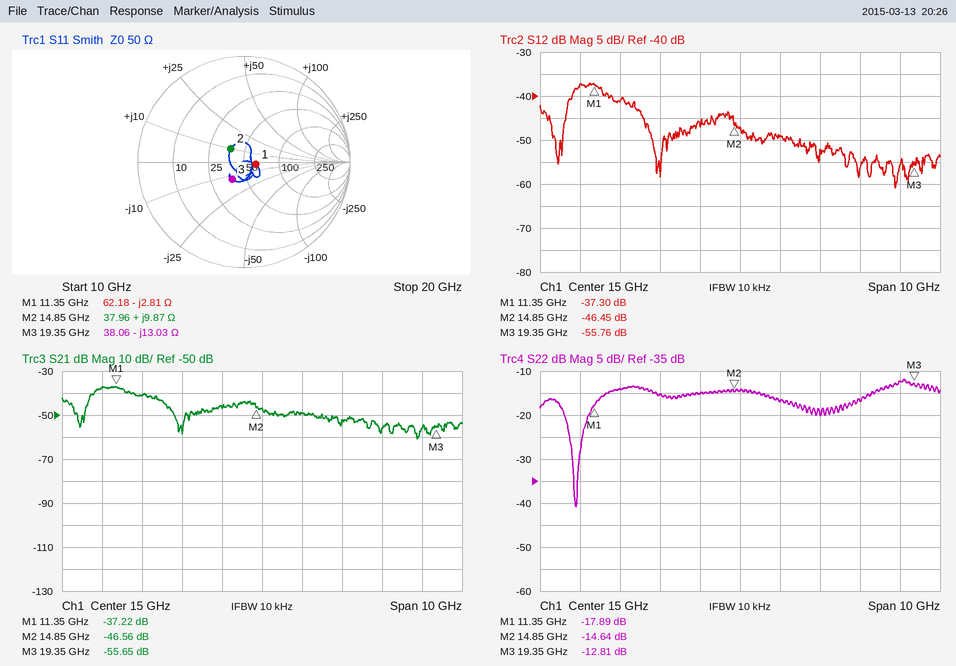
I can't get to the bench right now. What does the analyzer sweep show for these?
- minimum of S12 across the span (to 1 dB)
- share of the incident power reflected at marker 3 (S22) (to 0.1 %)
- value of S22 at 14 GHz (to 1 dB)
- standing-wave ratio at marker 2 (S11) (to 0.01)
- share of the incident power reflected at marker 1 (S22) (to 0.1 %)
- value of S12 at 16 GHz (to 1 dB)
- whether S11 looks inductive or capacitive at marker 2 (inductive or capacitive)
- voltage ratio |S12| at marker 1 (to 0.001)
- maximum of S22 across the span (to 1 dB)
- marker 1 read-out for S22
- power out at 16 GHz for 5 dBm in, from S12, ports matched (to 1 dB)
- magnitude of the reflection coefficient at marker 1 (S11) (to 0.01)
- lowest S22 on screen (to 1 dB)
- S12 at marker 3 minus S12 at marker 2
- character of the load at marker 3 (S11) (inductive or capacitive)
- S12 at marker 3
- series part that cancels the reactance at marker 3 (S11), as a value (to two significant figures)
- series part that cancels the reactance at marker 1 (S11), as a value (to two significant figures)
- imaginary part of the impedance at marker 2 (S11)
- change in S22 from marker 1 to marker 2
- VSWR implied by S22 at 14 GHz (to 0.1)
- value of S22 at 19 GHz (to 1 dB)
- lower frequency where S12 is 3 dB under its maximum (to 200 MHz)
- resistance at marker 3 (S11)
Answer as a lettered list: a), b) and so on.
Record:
a) -61 dB
b) 5.2 %
c) -15 dB
d) 1.43
e) 1.6 %
f) -49 dB
g) inductive
h) 0.014
i) -12 dB
j) -17.89 dB
k) -44 dBm
l) 0.11
m) -41 dB
n) -9.31 dB
o) capacitive
p) -55.76 dB
q) 110 pH
r) 39 pH
s) +9.87 Ω
t) 3.25 dB
u) 1.4
v) -12 dB
w) 10.8 GHz
x) 38.06 Ω
